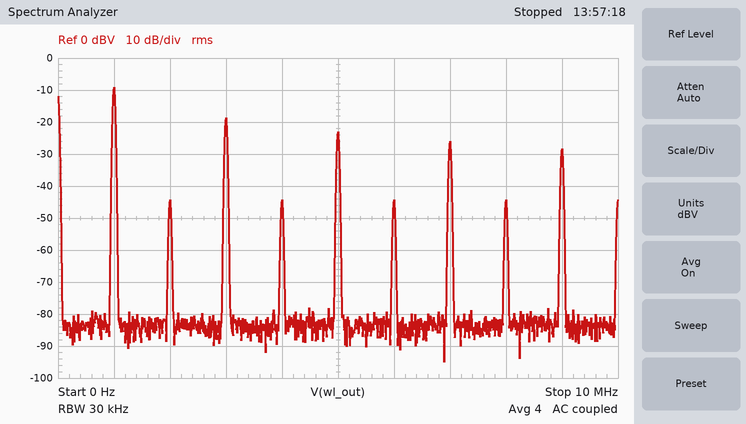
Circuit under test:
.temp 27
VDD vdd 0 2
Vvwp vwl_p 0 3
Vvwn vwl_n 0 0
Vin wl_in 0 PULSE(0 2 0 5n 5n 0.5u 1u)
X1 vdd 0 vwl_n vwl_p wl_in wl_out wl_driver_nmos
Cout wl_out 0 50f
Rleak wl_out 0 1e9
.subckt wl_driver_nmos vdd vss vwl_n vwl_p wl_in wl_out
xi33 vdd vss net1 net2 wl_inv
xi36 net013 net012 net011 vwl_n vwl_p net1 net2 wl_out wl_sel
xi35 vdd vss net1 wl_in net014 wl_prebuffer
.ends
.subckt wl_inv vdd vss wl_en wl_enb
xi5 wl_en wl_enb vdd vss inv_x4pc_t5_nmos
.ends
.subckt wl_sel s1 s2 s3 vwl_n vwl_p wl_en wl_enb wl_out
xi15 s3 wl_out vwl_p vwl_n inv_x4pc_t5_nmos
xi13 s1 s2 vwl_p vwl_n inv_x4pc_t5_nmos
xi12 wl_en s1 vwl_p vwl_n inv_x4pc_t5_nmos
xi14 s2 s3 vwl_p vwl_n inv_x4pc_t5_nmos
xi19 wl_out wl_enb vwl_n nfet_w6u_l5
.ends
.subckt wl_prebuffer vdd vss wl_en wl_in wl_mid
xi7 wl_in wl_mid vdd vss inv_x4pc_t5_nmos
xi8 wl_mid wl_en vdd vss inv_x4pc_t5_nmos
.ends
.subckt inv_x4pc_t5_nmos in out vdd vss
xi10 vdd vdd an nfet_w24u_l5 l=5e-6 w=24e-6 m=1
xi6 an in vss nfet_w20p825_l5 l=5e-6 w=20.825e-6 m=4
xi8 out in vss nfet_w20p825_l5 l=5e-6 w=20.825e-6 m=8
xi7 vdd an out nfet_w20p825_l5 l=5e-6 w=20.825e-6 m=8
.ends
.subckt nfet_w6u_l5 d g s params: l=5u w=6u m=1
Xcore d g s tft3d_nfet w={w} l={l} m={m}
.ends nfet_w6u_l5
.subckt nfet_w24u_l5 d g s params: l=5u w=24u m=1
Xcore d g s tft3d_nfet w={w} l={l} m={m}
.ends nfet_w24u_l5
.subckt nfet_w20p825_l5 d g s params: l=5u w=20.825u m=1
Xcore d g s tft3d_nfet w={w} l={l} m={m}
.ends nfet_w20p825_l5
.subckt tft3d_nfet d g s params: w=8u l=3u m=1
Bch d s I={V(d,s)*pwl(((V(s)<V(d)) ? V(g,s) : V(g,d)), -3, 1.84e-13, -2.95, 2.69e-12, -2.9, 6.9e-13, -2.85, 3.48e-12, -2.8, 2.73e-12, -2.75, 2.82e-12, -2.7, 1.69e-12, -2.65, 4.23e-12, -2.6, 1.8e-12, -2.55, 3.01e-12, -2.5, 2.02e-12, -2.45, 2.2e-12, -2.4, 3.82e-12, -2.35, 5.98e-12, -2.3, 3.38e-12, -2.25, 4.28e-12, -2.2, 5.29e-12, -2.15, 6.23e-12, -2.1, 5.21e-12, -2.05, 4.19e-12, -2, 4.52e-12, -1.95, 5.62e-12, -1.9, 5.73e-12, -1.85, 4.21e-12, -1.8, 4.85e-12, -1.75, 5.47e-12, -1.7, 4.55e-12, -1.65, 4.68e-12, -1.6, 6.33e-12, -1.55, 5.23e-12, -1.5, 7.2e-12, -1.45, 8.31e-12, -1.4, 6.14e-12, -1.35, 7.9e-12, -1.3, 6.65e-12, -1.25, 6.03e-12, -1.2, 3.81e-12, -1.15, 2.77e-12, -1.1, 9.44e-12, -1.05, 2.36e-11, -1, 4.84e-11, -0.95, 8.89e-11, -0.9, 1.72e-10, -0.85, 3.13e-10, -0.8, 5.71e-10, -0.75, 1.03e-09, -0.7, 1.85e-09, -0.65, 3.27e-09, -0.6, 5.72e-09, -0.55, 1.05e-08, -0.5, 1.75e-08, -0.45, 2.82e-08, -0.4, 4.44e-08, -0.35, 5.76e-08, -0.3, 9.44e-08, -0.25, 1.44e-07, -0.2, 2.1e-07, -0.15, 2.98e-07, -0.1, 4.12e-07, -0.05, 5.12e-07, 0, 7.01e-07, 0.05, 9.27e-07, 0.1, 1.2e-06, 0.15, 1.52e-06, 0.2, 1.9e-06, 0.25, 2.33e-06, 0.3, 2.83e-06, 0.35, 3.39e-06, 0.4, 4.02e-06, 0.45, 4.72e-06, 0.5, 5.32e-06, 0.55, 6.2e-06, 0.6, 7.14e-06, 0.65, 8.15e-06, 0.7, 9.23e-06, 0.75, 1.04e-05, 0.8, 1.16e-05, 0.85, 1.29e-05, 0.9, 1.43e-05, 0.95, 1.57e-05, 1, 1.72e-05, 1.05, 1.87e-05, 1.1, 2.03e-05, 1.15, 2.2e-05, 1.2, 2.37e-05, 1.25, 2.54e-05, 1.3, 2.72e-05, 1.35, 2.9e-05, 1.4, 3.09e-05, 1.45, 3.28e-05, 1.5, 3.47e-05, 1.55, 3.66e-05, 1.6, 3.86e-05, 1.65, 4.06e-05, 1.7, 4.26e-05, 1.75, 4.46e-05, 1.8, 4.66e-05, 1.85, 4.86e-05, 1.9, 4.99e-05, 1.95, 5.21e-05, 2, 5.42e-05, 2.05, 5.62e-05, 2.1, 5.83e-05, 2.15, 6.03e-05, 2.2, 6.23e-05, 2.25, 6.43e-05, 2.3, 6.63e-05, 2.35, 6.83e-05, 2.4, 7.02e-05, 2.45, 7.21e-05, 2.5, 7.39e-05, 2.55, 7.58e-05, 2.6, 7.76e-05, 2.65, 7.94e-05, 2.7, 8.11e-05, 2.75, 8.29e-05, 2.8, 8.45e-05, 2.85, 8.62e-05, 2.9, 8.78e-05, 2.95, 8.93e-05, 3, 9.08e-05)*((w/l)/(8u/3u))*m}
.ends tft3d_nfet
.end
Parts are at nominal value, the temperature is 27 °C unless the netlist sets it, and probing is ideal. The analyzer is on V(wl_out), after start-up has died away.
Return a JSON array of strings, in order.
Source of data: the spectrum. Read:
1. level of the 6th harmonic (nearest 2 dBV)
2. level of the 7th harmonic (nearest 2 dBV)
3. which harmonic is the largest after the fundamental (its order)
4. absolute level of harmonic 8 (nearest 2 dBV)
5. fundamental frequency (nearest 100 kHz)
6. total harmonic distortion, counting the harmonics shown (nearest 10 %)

["-44 dBV", "-26 dBV", "3", "-44 dBV", "1.0 MHz", "40 %"]
